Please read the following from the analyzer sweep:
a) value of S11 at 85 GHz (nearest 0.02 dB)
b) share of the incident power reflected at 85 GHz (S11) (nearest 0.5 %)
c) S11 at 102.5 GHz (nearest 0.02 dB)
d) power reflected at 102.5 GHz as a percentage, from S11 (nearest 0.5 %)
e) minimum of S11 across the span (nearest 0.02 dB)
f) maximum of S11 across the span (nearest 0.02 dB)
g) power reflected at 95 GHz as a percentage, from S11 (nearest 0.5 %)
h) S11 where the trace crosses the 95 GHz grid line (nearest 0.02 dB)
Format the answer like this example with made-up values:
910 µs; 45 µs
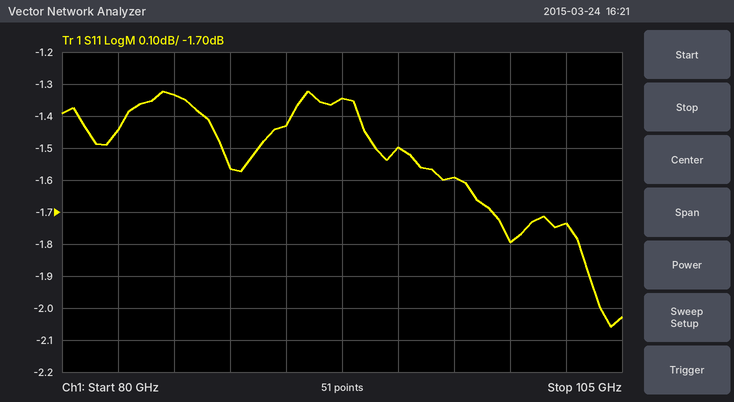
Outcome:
-1.34 dB; 73.5 %; -1.74 dB; 67.0 %; -2.06 dB; -1.32 dB; 71.0 %; -1.50 dB
